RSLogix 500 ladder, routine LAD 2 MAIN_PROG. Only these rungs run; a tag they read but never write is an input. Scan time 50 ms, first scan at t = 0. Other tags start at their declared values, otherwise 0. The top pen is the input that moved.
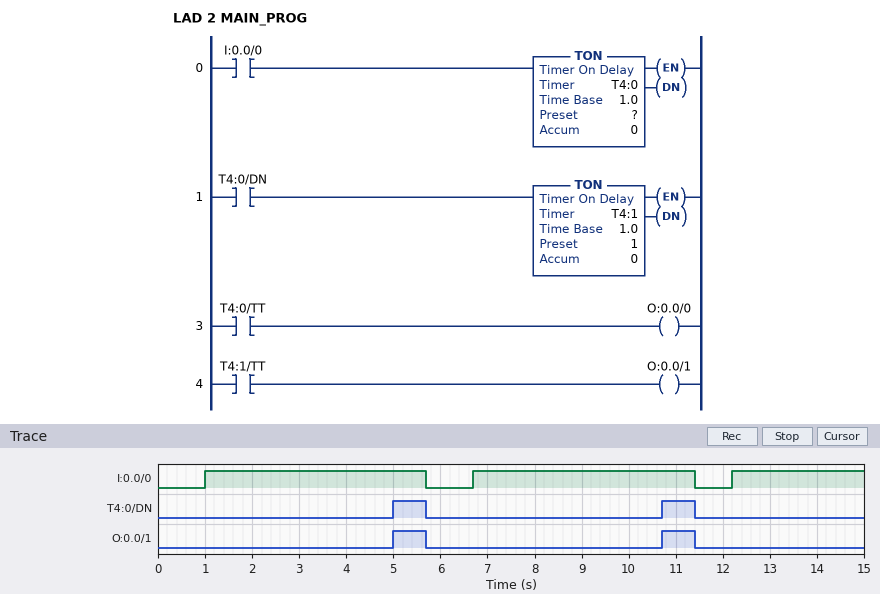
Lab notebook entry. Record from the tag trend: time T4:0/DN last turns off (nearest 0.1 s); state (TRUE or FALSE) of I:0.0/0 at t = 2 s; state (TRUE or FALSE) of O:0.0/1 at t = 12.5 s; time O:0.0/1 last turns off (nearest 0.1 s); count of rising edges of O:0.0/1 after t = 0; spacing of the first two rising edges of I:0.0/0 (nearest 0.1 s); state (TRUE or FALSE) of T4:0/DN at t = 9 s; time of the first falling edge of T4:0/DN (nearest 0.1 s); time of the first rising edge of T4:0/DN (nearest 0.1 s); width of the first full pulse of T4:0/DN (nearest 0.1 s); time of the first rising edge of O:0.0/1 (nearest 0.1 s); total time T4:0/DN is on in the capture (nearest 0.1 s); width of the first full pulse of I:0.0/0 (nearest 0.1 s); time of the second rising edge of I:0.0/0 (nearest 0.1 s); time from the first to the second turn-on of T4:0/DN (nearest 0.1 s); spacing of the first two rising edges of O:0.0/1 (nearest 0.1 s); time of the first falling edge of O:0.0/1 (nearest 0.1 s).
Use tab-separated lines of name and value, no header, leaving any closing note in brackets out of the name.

time T4:0/DN last turns off	11.4 s
state (TRUE or FALSE) of I:0.0/0 at t = 2 s	TRUE
state (TRUE or FALSE) of O:0.0/1 at t = 12.5 s	FALSE
time O:0.0/1 last turns off	11.4 s
count of rising edges of O:0.0/1 after t = 0	2
spacing of the first two rising edges of I:0.0/0	5.7 s
state (TRUE or FALSE) of T4:0/DN at t = 9 s	FALSE
time of the first falling edge of T4:0/DN	5.7 s
time of the first rising edge of T4:0/DN	5.0 s
width of the first full pulse of T4:0/DN	0.7 s
time of the first rising edge of O:0.0/1	5.0 s
total time T4:0/DN is on in the capture	1.4 s
width of the first full pulse of I:0.0/0	4.7 s
time of the second rising edge of I:0.0/0	6.7 s
time from the first to the second turn-on of T4:0/DN	5.7 s
spacing of the first two rising edges of O:0.0/1	5.7 s
time of the first falling edge of O:0.0/1	5.7 s
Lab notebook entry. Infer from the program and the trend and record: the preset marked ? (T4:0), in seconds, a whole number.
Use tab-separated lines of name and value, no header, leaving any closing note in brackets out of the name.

the preset marked ? (T4:0), in seconds, a whole number	4 s
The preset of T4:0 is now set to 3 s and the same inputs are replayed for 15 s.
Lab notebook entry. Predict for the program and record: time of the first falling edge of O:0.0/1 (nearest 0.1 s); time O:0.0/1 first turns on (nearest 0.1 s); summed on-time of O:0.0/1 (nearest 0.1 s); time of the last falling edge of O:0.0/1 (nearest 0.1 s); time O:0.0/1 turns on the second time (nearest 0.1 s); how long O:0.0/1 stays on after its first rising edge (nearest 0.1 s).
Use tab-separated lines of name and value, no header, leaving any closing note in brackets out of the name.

time of the first falling edge of O:0.0/1	5.0 s
time O:0.0/1 first turns on	4.0 s
summed on-time of O:0.0/1	2.0 s
time of the last falling edge of O:0.0/1	10.7 s
time O:0.0/1 turns on the second time	9.7 s
how long O:0.0/1 stays on after its first rising edge	1.0 s
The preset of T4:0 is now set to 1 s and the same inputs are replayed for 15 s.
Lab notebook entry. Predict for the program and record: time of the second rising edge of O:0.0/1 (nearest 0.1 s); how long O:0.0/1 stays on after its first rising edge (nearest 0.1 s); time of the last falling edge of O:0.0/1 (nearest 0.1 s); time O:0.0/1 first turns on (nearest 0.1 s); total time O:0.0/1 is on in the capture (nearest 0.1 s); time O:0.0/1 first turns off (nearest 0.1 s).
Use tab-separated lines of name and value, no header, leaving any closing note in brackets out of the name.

time of the second rising edge of O:0.0/1	7.7 s
how long O:0.0/1 stays on after its first rising edge	1.0 s
time of the last falling edge of O:0.0/1	14.2 s
time O:0.0/1 first turns on	2.0 s
total time O:0.0/1 is on in the capture	3.0 s
time O:0.0/1 first turns off	3.0 s
